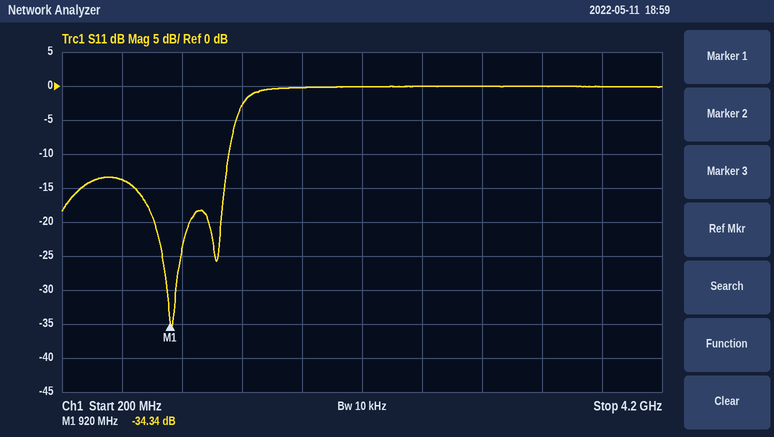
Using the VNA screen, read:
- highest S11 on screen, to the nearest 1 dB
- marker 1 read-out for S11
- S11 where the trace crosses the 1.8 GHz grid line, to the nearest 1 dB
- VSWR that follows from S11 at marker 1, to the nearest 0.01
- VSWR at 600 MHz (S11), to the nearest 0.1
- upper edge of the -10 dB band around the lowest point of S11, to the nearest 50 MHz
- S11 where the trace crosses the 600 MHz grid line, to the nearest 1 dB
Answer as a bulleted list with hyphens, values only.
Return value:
- 0 dB
- -34.34 dB
- 0 dB
- 1.04
- 1.5
- 1.30 GHz
- -14 dB
